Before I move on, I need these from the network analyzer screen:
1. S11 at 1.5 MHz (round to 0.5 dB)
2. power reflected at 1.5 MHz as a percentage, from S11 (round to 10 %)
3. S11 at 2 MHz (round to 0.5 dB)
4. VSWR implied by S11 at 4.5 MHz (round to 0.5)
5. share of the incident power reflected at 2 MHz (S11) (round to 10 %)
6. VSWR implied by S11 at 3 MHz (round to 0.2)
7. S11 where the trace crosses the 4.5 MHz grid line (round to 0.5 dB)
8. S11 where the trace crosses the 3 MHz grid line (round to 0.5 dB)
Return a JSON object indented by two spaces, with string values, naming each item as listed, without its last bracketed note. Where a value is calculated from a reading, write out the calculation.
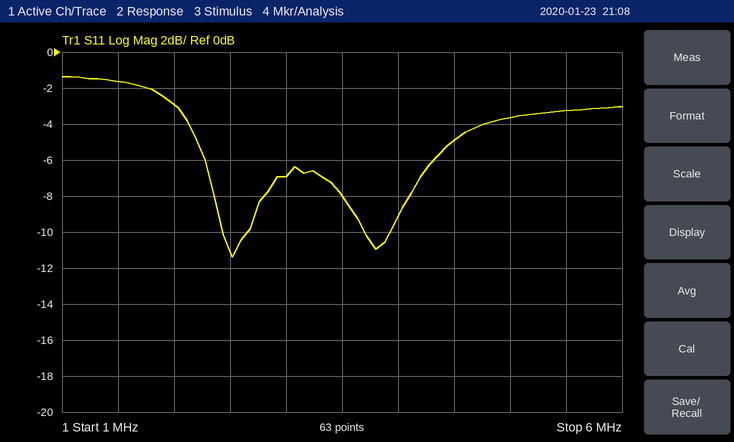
{
  "S11 at 1.5 MHz": "-1.5 dB",
  "power reflected at 1.5 MHz as a percentage, from S11": "10^(-1.5/10) ≈ 70.8 %, so 70 % to the nearest 10 %",
  "S11 at 2 MHz": "-3.0 dB",
  "VSWR implied by S11 at 4.5 MHz": "|Γ| = 10^(-5/20) = 0.5623; VSWR = (1 + 0.5623)/(1 − 0.5623) ≈ 3.57, so 3.5 to the nearest 0.5",
  "share of the incident power reflected at 2 MHz (S11)": "10^(-3/10) ≈ 50 %",
  "VSWR implied by S11 at 3 MHz": "|Γ| = 10^(-7/20) = 0.4467; VSWR = (1 + 0.4467)/(1 − 0.4467) ≈ 2.6",
  "S11 where the trace crosses the 4.5 MHz grid line": "-5.0 dB",
  "S11 where the trace crosses the 3 MHz grid line": "-7.0 dB"
}
